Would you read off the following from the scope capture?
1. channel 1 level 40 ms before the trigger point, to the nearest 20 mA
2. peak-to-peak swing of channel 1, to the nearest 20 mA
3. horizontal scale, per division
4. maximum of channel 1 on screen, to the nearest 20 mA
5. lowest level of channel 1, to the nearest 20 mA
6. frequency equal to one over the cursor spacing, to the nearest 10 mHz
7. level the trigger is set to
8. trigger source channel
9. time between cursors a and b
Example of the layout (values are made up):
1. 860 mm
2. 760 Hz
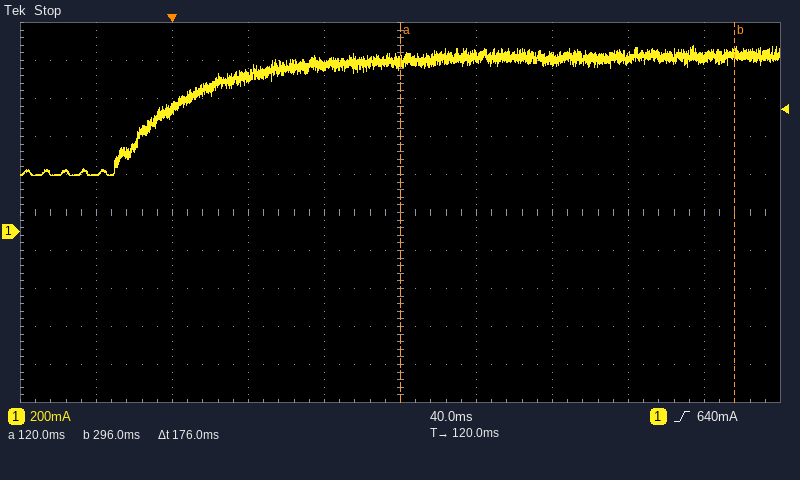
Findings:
1. 300 mA
2. 680 mA
3. 40 ms
4. 980 mA
5. 300 mA
6. 5.68 Hz
7. 640 mA
8. channel 1
9. 176 ms
